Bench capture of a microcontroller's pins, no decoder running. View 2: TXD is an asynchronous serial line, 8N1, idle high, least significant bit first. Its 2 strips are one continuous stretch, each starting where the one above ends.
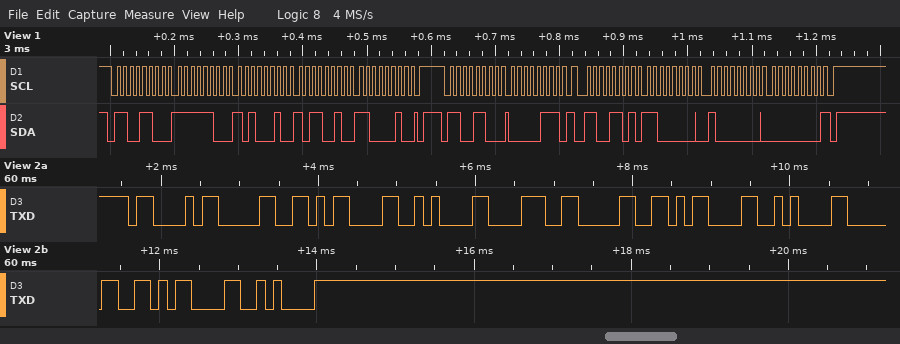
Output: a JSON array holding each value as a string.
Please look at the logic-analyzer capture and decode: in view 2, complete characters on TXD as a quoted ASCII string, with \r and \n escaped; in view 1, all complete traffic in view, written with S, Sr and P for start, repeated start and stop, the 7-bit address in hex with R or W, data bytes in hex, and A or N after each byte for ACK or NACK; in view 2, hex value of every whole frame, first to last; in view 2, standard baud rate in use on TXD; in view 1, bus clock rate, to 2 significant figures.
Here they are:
["\"C0\\r\\n80\\r\\n0\\r\\n\"", "S 66W A FC A A2 A B2 A C2 A P S 66W A 07 A Sr 66R A C0 A 80 A 00 N P", "0x43 0x30 0x0D 0x0A 0x38 0x30 0x0D 0x0A 0x30 0x0D 0x0A", "9600 baud", "100 kHz"]
